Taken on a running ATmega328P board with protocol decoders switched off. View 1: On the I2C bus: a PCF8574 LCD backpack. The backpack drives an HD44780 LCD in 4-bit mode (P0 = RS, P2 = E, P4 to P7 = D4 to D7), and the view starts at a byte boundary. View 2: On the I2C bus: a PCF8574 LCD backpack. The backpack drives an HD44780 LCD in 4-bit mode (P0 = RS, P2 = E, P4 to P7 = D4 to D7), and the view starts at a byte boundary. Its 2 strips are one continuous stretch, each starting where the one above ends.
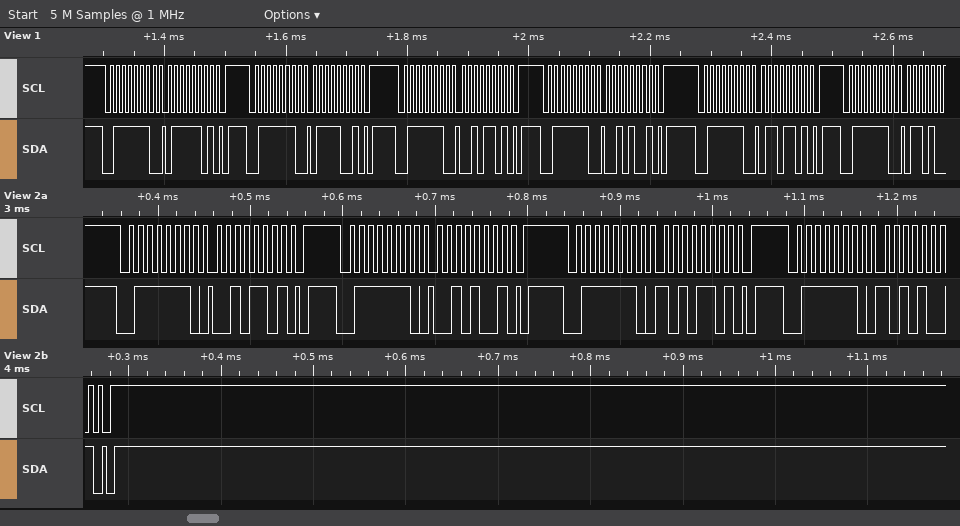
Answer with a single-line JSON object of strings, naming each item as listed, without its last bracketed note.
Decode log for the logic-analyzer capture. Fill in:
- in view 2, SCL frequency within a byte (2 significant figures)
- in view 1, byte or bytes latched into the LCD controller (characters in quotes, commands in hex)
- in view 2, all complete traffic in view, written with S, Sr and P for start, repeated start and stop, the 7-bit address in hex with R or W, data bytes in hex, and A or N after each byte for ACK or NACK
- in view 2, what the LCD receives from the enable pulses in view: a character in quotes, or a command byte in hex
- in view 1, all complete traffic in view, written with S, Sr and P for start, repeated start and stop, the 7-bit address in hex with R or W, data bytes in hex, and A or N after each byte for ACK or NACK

{"in view 2, SCL frequency within a byte": "100 kHz", "in view 1, byte or bytes latched into the LCD controller": "'r'", "in view 2, all complete traffic in view, written with S, Sr and P for start, repeated start and stop, the 7-bit address in hex with R or W, data bytes in hex, and A or N after each byte for ACK or NACK": "S 3FW A 2D A P S 3FW A 29 A P S 3FW A AD A P S 3FW A A9 A P", "in view 2, what the LCD receives from the enable pulses in view: a character in quotes, or a command byte in hex": "'*'", "in view 1, all complete traffic in view, written with S, Sr and P for start, repeated start and stop, the 7-bit address in hex with R or W, data bytes in hex, and A or N after each byte for ACK or NACK": "S 3FW A 7D A P S 3FW A 79 A P S 3FW A 2D A P S 3FW A 29 A P S 3FW A 6D A P S 3FW A"}
